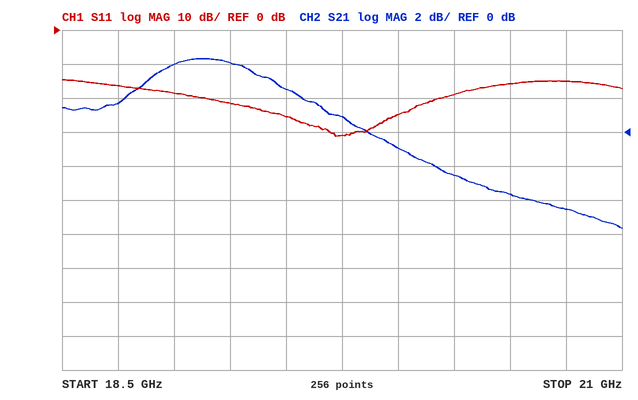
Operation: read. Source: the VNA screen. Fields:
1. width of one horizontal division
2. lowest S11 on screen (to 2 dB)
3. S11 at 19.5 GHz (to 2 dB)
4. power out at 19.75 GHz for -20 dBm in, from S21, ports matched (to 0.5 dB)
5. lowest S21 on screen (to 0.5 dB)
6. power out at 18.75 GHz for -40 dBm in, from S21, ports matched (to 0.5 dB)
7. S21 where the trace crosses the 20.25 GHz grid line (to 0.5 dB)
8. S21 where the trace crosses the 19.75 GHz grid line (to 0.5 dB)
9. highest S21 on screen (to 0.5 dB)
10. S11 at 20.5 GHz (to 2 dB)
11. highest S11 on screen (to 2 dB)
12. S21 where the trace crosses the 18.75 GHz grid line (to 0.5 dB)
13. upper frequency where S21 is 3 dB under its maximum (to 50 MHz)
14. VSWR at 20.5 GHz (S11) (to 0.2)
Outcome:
250 MHz
-32 dB
-26 dB
-19.0 dBm
-5.5 dB
-38.5 dBm
-2.5 dB
1.0 dB
4.5 dB
-16 dB
-14 dB
1.5 dB
19.65 GHz
1.4
